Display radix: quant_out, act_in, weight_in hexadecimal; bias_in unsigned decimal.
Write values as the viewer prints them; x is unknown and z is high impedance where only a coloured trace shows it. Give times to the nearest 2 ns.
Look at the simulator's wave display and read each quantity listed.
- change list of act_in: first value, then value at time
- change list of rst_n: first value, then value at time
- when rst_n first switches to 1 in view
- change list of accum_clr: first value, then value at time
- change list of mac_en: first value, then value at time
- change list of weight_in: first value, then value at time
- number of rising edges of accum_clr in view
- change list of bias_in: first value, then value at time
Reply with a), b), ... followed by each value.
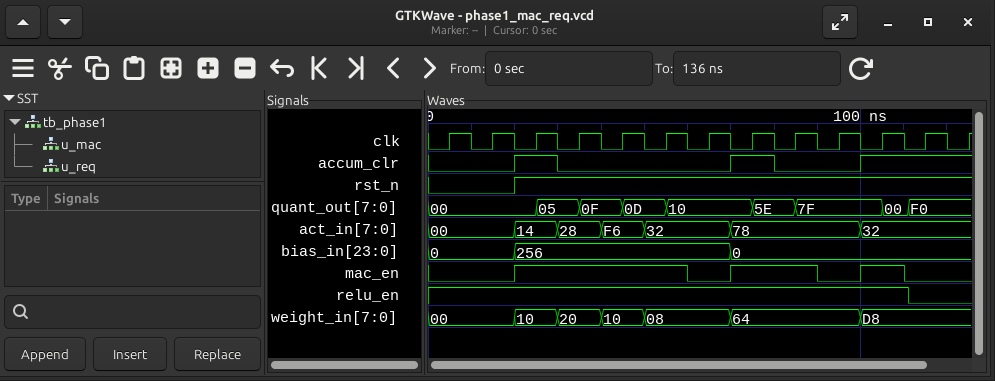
a) 00, 14 at 20 ns, 28 at 30 ns, F6 at 40 ns, 32 at 50 ns, 78 at 70 ns, 32 at 100 ns
b) 0, 1 at 20 ns
c) 20 ns
d) 0, 1 at 20 ns, 0 at 30 ns, 1 at 70 ns, 0 at 80 ns, 1 at 100 ns
e) 0, 1 at 20 ns, 0 at 60 ns, 1 at 70 ns, 0 at 90 ns, 1 at 100 ns, 0 at 110 ns
f) 00, 10 at 20 ns, 20 at 30 ns, 10 at 40 ns, 08 at 50 ns, 64 at 70 ns, D8 at 100 ns
g) 3
h) 0, 256 at 20 ns, 0 at 70 ns
